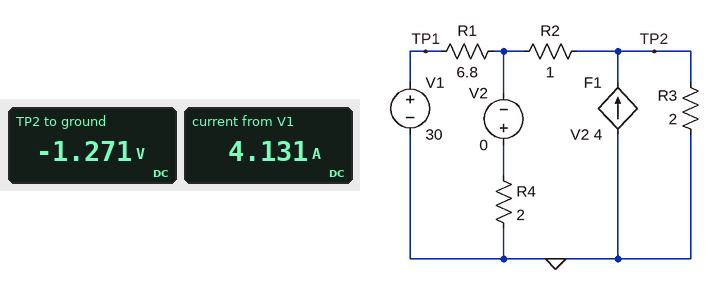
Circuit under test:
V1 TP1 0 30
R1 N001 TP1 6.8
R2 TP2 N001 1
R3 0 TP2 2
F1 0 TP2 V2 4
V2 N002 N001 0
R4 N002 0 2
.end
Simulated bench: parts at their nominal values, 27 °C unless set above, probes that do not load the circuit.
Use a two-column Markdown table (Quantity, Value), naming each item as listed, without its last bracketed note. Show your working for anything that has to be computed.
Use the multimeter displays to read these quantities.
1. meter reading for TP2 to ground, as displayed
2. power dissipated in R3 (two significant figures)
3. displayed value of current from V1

| Quantity | Value |
|---|---|
| meter reading for TP2 to ground, as displayed | -1.271 V |
| power dissipated in R3 | (0 V - (-1.271 V))^2 / 2 Ω = 810 mW |
| displayed value of current from V1 | 4.131 A |
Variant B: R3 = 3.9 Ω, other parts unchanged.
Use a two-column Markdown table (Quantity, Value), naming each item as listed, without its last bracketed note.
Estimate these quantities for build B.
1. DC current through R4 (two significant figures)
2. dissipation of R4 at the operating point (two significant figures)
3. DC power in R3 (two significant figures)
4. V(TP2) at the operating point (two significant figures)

| Quantity | Value |
|---|---|
| DC current through R4 | 900 mA |
| dissipation of R4 at the operating point | 1.6 W |
| DC power in R3 | 530 mW |
| V(TP2) at the operating point | -1.4 V |
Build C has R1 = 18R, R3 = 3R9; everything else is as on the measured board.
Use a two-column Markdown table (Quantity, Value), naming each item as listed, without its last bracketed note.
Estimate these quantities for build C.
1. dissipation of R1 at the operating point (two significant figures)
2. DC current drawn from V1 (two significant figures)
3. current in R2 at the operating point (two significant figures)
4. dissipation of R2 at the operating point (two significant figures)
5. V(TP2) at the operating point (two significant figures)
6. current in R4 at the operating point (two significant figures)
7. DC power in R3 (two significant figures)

| Quantity | Value |
|---|---|
| dissipation of R1 at the operating point | 48 W |
| DC current drawn from V1 | 1.6 A |
| current in R2 at the operating point | 1.3 A |
| dissipation of R2 at the operating point | 1.6 W |
| V(TP2) at the operating point | -560 mV |
| current in R4 at the operating point | 350 mA |
| DC power in R3 | 82 mW |
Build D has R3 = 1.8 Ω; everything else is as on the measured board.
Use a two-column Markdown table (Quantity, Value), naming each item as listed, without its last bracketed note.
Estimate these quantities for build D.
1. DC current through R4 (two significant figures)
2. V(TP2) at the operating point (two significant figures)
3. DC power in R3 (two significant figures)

| Quantity | Value |
|---|---|
| DC current through R4 | 960 mA |
| V(TP2) at the operating point | -1.2 V |
| DC power in R3 | 850 mW |
